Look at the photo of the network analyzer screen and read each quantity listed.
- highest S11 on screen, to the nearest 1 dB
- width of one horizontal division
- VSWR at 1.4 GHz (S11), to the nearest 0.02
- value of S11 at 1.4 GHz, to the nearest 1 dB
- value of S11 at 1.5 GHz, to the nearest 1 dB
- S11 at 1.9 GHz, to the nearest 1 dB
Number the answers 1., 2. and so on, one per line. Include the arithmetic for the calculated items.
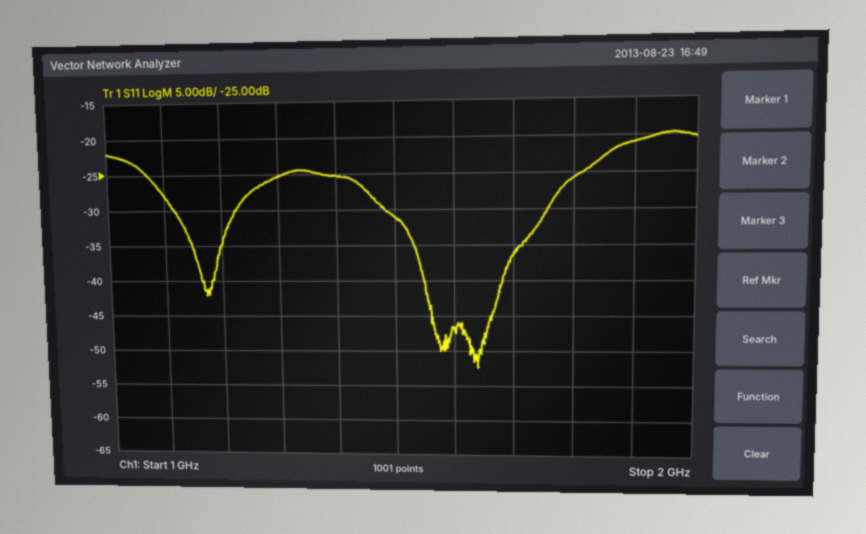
1. -20 dB
2. 100 MHz
3. |Γ| = 10^(-25/20) = 0.0562; VSWR = (1 + 0.0562)/(1 − 0.0562) ≈ 1.12
4. -25 dB
5. -31 dB
6. -21 dB
